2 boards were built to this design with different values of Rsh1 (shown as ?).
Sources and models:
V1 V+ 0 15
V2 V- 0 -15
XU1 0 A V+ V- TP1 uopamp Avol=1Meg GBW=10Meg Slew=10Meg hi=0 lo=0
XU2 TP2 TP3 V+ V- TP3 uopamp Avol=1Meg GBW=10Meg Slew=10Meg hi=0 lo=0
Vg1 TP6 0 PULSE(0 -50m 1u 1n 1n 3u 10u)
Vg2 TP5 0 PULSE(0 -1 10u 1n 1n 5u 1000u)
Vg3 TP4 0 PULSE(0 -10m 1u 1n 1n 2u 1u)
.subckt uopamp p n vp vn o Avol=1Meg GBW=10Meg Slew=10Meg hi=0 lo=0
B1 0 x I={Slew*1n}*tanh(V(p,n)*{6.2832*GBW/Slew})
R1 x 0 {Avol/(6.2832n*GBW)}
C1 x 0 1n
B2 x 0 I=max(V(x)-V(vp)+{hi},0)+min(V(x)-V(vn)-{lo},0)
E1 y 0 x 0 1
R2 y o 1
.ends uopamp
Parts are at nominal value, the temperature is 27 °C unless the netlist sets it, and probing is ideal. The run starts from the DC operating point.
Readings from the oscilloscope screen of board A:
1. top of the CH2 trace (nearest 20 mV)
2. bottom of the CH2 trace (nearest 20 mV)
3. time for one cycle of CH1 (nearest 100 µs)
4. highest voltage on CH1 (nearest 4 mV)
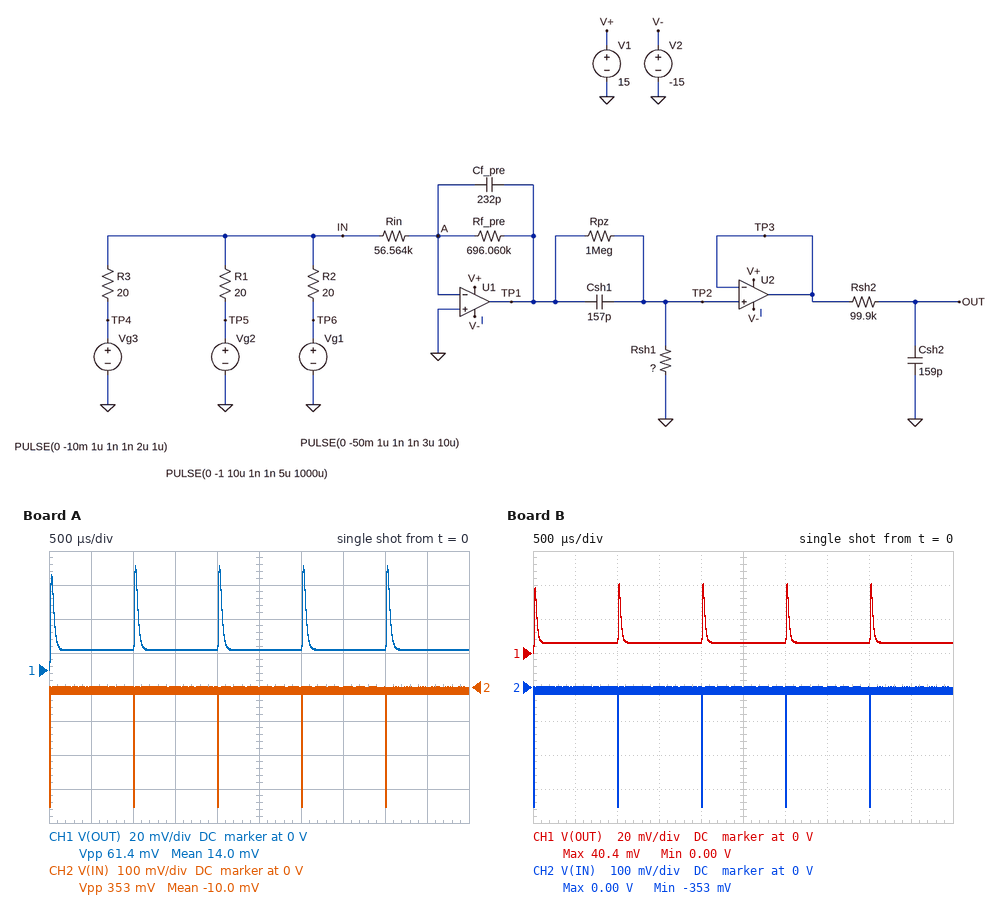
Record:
0 V
-360 mV
1.0 ms
60 mV
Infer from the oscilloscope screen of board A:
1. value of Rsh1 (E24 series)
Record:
130 kΩ
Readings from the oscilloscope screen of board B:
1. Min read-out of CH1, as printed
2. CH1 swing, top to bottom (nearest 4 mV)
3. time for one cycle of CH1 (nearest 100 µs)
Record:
0.00 V
40 mV
1.0 ms
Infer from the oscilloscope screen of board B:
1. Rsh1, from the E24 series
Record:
62 kΩ
